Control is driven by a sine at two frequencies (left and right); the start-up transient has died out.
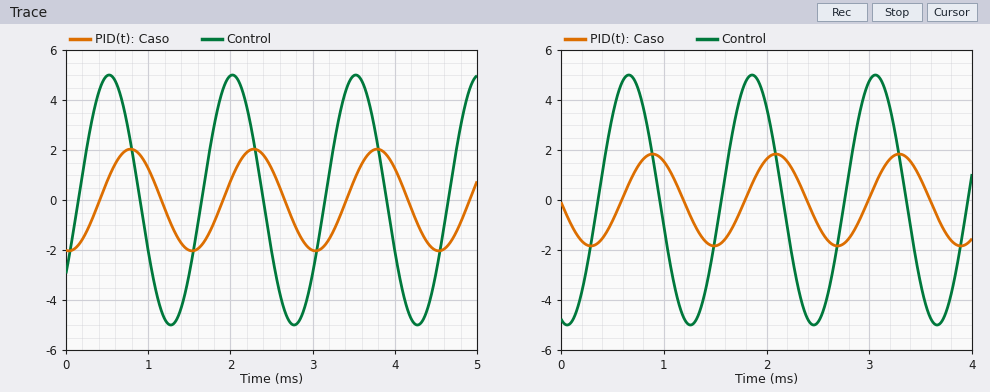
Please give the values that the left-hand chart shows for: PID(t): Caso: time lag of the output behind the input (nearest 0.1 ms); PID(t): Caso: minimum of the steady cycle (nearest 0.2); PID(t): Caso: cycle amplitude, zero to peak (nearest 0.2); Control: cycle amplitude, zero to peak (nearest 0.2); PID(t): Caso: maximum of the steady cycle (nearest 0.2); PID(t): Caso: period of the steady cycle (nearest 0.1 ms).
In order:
0.3 ms
-2.0
2.0
5.0
2.0
1.5 ms
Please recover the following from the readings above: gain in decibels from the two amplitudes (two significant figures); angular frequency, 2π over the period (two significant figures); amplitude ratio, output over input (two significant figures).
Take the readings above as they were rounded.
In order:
-8.0 dB
4.2 rad/ms
0.40
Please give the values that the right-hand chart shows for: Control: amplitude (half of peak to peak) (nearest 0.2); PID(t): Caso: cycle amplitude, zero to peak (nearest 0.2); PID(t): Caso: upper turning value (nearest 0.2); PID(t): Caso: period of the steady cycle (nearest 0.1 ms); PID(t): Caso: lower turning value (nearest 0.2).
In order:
5.0
1.8
1.8
1.2 ms
-1.8
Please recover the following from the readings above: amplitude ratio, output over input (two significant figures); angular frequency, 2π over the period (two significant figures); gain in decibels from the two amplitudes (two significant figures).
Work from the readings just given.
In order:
0.36
5.2 rad/ms
-8.9 dB
